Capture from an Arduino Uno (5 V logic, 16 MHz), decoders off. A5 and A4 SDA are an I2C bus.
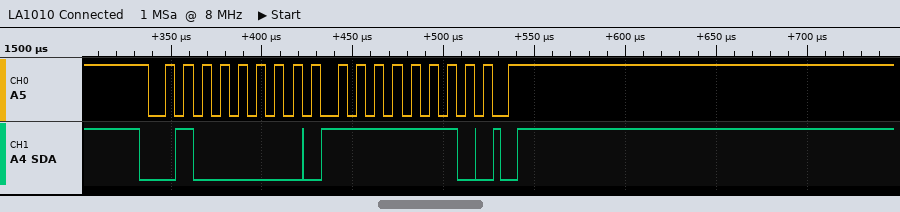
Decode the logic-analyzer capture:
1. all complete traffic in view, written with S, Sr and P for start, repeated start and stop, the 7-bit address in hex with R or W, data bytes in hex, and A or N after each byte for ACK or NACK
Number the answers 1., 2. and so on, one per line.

1. S 20W A FE A P
